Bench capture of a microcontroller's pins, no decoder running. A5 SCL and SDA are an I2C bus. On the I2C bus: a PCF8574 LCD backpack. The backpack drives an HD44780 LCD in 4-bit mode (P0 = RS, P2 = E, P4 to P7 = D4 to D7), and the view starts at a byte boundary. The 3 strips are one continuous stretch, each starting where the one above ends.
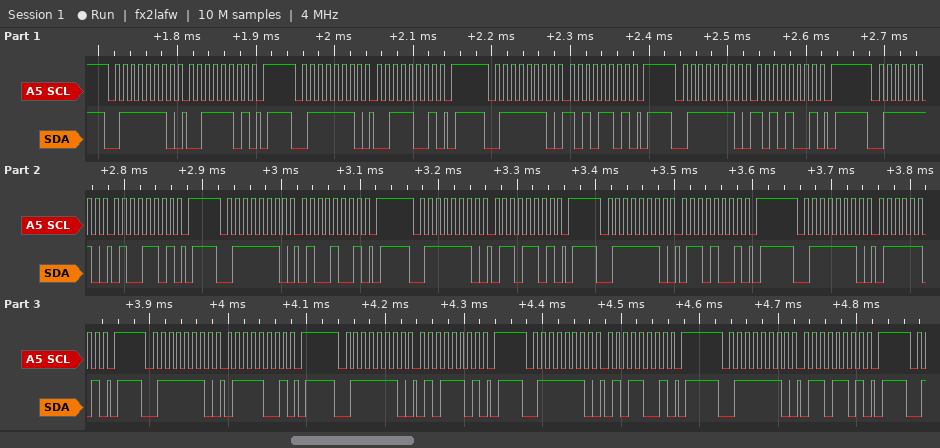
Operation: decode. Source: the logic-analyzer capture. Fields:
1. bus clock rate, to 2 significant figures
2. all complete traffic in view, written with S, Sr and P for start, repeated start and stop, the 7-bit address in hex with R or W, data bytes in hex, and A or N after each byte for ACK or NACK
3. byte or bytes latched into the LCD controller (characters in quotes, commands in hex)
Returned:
100 kHz
S 3FW A 3D A P S 3FW A 39 A P S 3FW A AD A P S 3FW A A9 A P S 3FW A 4D A P S 3FW A 49 A P S 3FW A 6D A P S 3FW A 69 A P S 3FW A 7D A P S 3FW A 79 A P S 3FW A 5D A P S 3FW A 59 A P S 3FW A 6D A P
':' 'F' 'u'
